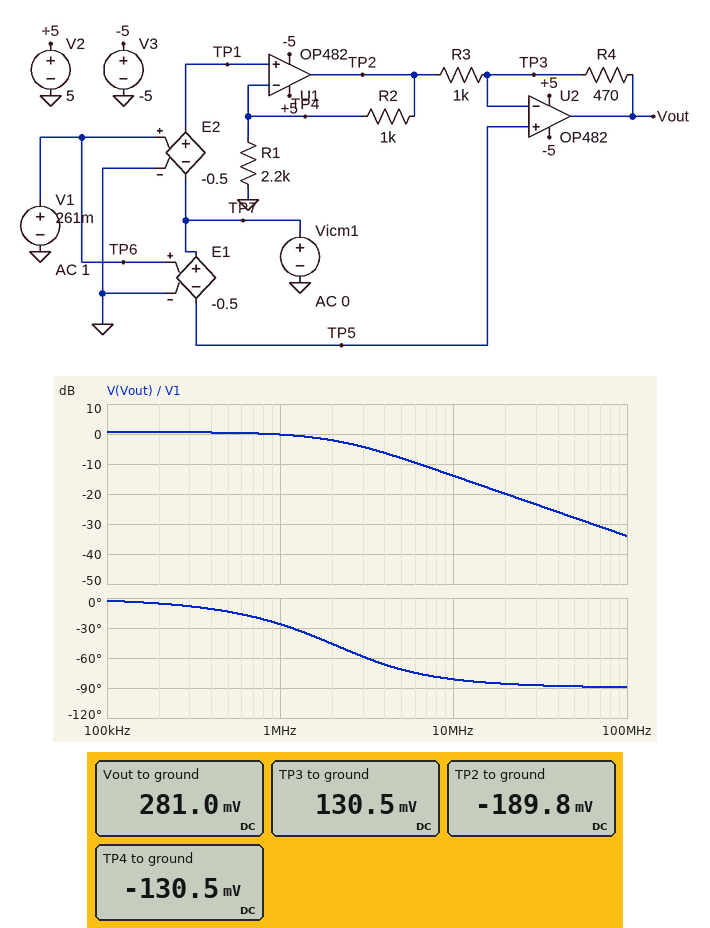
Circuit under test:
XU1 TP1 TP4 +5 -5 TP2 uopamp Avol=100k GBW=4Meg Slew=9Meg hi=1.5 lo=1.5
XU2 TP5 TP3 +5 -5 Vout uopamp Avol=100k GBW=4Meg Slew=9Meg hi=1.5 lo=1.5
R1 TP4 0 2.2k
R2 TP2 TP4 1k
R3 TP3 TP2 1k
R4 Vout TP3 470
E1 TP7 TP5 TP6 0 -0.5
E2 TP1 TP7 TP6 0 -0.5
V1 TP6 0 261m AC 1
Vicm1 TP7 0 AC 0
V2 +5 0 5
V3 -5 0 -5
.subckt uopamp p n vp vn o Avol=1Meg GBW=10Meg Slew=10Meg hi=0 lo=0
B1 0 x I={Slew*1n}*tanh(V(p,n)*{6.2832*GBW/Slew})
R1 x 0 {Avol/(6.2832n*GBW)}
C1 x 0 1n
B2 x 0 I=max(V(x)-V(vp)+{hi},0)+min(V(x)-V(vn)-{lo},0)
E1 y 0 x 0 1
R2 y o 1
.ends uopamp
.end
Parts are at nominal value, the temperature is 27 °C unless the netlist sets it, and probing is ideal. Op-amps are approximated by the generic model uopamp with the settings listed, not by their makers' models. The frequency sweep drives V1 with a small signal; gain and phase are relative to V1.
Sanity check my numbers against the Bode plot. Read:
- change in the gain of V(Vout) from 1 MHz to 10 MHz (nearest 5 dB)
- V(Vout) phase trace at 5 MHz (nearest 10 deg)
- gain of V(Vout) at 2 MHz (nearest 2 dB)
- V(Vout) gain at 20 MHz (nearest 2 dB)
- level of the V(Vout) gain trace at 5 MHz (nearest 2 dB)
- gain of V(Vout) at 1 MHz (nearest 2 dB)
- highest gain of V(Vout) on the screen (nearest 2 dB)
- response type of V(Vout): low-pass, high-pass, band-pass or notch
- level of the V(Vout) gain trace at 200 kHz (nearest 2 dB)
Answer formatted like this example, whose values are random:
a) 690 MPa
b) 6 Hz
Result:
a) -15 dB
b) -70 deg
c) -2 dB
d) -20 dB
e) -8 dB
f) 0 dB
g) 0 dB
h) low-pass
i) 0 dB
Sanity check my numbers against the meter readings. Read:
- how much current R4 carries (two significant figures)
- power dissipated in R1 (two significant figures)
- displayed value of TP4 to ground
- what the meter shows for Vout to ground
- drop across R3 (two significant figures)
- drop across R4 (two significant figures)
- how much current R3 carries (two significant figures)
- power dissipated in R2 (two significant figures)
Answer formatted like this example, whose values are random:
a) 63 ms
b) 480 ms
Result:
a) 320 µA
b) 7.7 µW
c) -130.5 mV
d) 281.0 mV
e) 320 mV
f) 150 mV
g) 320 µA
h) 3.5 µW
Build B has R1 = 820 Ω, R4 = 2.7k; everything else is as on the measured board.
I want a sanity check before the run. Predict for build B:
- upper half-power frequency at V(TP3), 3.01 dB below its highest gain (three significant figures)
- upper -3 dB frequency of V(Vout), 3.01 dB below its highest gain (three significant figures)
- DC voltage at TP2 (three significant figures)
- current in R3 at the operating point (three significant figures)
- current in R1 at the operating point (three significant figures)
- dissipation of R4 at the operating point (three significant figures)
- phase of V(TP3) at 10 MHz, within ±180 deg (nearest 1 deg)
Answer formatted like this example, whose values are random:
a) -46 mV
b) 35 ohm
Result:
a) 1.85 MHz
b) 883 kHz
c) -290 mV
d) 420 µA
e) 159 µA
f) 477 µW
g) 112 deg
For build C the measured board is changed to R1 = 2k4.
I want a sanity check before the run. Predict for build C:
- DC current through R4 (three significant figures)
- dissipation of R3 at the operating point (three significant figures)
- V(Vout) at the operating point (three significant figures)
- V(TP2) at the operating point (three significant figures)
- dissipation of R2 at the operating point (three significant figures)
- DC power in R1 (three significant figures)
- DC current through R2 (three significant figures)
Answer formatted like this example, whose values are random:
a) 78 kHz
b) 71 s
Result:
a) 315 µA
b) 99.5 µW
c) 279 mV
d) -185 mV
e) 2.96 µW
f) 7.10 µW
g) 54.4 µA
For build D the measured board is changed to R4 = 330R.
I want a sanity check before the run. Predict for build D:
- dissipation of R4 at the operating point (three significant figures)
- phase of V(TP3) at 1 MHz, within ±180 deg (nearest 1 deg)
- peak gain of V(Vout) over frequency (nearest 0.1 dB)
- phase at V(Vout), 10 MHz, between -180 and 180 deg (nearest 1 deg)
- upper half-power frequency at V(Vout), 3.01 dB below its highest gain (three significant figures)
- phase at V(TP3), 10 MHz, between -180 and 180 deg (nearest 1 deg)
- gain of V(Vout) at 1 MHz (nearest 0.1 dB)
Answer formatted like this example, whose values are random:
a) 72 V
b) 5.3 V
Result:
a) 33.9 µW
b) -25 deg
c) -0.9 dB
d) -78 deg
e) 2.35 MHz
f) -80 deg
g) -1.6 dB
